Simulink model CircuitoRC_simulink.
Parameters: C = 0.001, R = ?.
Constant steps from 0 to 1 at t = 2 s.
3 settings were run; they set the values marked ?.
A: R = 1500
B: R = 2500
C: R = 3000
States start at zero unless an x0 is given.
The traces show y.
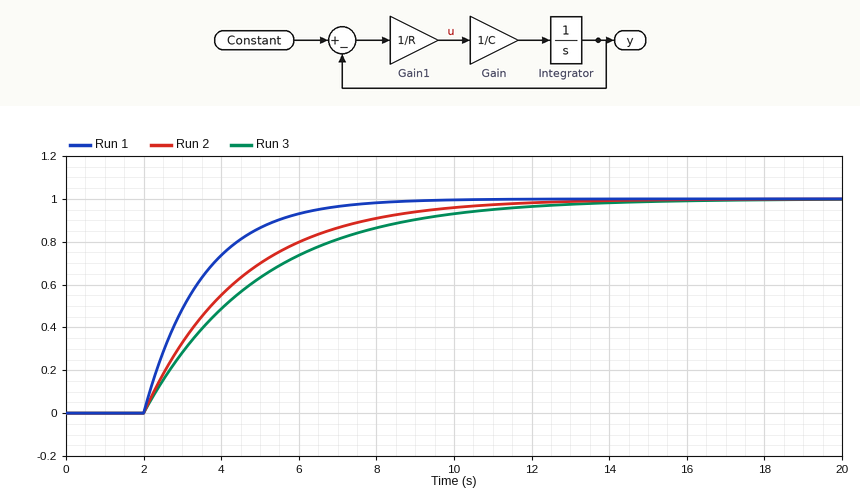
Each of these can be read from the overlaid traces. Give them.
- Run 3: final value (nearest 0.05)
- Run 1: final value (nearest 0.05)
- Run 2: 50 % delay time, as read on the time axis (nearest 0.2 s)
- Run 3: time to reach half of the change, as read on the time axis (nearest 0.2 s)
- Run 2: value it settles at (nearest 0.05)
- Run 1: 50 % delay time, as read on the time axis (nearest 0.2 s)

1.00
1.00
3.8 s
4.0 s
1.00
3.0 s
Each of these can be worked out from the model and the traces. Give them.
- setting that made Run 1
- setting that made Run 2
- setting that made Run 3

A
B
C
